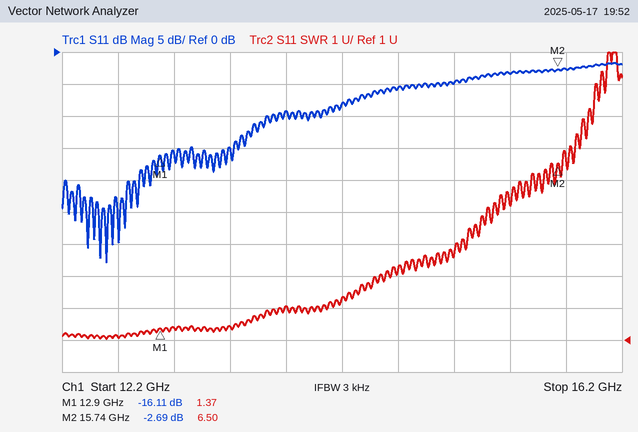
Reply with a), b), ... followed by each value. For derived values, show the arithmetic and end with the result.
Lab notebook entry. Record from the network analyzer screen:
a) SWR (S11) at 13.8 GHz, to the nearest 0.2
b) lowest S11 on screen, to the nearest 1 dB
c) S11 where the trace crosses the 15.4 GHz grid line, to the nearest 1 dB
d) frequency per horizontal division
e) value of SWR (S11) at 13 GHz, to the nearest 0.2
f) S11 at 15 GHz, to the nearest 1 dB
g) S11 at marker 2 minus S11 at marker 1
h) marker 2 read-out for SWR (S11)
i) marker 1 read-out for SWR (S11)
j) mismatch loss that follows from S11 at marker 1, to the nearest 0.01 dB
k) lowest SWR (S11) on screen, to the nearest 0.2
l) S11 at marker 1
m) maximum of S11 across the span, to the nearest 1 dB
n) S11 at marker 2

a) 2.0
b) -33 dB
c) -3 dB
d) 400 MHz
e) 1.4
f) -5 dB
g) -2.69 − (-16.11) = 13.42 dB
h) 6.50
i) 1.37
j) −10 log10(1 − 10^(-16.11/10)) ≈ 0.11 dB
k) 1.0
l) -16.11 dB
m) -2 dB
n) -2.69 dB
